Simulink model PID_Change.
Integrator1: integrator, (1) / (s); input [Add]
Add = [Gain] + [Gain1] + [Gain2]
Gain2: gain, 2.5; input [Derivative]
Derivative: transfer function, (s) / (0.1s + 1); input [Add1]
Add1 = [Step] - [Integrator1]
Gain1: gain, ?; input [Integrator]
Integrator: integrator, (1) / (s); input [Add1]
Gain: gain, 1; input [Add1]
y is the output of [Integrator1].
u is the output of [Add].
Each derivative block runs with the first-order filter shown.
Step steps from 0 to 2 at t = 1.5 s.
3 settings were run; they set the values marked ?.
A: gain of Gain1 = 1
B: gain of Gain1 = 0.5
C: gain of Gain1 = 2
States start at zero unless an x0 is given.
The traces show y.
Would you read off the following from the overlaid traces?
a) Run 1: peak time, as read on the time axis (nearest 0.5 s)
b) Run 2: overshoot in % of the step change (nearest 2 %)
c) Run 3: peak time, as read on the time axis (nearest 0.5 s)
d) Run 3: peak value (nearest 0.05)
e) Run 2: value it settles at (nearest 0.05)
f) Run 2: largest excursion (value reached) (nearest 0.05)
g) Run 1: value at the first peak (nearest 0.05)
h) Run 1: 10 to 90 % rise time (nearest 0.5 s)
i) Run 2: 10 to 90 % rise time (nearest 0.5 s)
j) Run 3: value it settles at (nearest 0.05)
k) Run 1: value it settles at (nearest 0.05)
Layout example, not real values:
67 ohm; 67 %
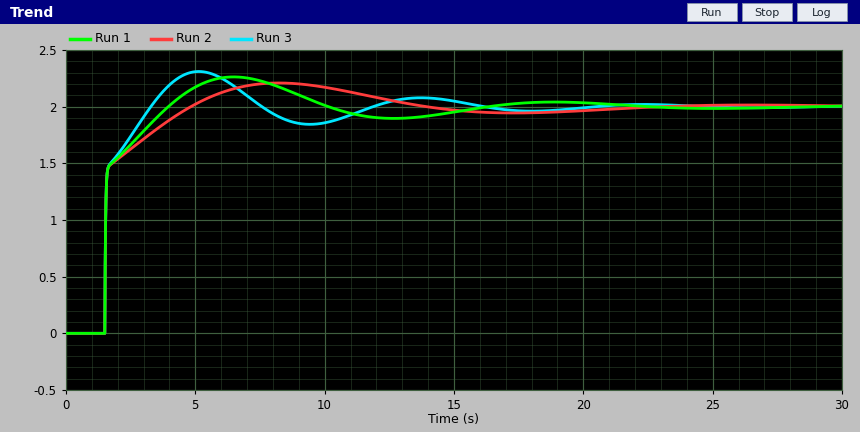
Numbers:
6.5 s; 10 %; 5.0 s; 2.30; 2.00; 2.20; 2.25; 1.5 s; 2.0 s; 2.00; 2.00
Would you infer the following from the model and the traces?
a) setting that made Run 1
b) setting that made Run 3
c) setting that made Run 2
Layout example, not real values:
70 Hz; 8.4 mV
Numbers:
A; C; B
